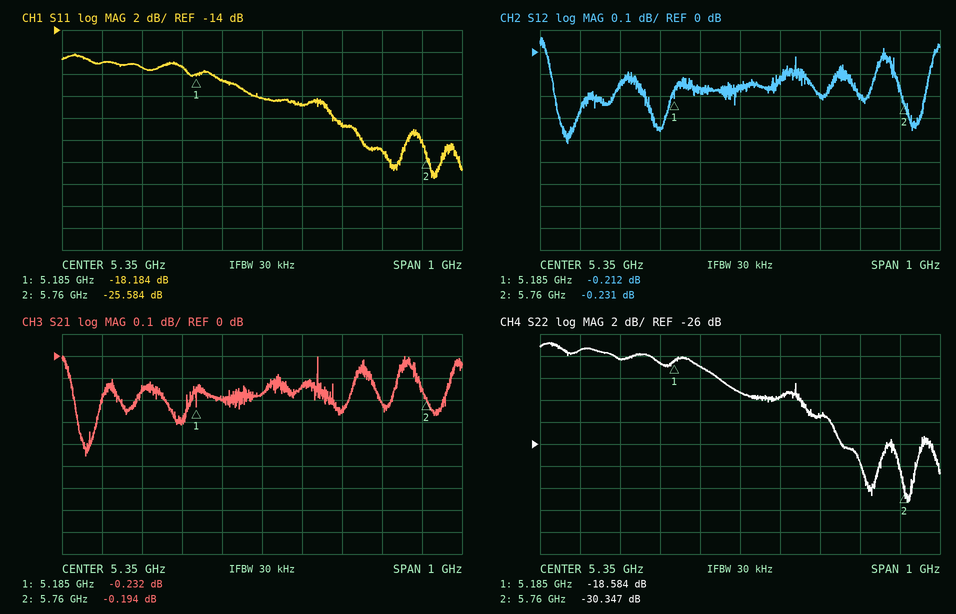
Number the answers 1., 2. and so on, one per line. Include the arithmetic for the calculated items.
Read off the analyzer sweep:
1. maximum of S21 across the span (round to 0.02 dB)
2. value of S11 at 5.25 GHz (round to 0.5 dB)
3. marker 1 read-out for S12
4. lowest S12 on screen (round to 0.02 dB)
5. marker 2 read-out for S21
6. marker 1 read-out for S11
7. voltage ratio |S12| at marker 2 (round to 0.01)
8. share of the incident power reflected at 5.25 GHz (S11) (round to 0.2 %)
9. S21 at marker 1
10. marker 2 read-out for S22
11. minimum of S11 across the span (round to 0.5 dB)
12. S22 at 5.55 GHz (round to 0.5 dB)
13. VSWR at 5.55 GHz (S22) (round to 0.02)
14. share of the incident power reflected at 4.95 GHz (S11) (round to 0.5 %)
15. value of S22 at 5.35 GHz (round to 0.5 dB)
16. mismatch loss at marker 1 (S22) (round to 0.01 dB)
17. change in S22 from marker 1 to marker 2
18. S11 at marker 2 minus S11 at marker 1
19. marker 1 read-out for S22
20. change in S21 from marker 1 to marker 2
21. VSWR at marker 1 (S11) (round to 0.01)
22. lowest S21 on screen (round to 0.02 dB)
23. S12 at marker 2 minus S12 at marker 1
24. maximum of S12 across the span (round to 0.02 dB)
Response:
1. 0.00 dB
2. -18.5 dB
3. -0.212 dB
4. -0.42 dB
5. -0.194 dB
6. -18.184 dB
7. 10^(-0.231/20) ≈ 0.97
8. 10^(-18.5/10) ≈ 1.4 %
9. -0.232 dB
10. -30.347 dB
11. -27.5 dB
12. -23.5 dB
13. |Γ| = 10^(-23.5/20) = 0.0668; VSWR = (1 + 0.0668)/(1 − 0.0668) ≈ 1.14
14. 10^(-17/10) ≈ 2.0 %
15. -21.5 dB
16. −10 log10(1 − 10^(-18.584/10)) ≈ 0.06 dB
17. -30.347 − (-18.584) = -11.763 dB
18. -25.584 − (-18.184) = -7.400 dB
19. -18.584 dB
20. -0.194 − (-0.232) = 0.038 dB
21. (1 + 0.1233)/(1 − 0.1233) ≈ 1.28
22. -0.46 dB
23. -0.231 − (-0.212) = -0.019 dB
24. 0.06 dB
